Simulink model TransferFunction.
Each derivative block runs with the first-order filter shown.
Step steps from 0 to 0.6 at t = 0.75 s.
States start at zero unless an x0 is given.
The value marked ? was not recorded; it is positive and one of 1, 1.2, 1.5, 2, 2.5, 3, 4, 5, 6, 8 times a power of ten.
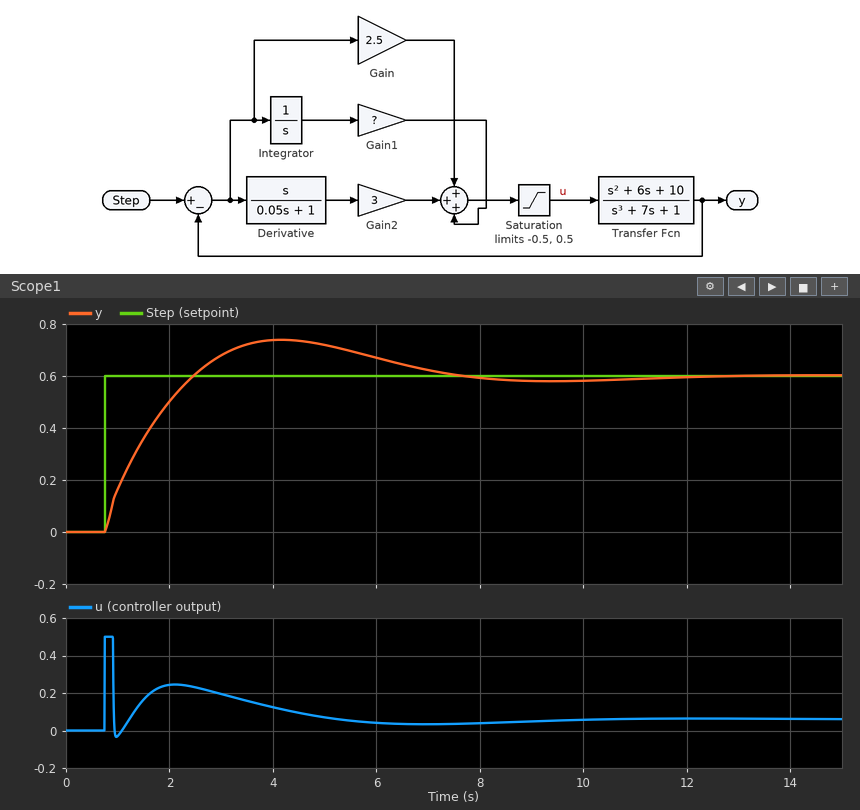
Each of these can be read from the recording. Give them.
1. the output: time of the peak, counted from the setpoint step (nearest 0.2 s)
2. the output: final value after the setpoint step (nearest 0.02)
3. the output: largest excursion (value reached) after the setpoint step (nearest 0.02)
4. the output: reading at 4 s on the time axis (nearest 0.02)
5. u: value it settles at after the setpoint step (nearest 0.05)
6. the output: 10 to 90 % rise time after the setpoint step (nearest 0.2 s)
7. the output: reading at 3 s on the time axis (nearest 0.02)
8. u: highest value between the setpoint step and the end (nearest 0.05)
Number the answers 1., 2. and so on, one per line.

1. 3.4 s
2. 0.60
3. 0.74
4. 0.74
5. 0.05
6. 1.4 s
7. 0.68
8. 0.50
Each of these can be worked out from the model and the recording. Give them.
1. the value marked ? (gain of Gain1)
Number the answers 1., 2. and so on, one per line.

1. 2
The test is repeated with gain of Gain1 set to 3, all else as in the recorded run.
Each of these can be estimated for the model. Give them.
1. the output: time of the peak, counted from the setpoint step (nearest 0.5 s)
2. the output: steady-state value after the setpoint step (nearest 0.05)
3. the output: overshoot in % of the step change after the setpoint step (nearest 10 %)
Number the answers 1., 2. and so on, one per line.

1. 3.0 s
2. 0.60
3. 30 %
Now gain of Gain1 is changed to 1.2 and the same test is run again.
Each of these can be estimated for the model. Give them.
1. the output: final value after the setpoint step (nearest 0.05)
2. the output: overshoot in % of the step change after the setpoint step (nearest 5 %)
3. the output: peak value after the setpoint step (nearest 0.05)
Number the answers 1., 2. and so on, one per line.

1. 0.60
2. 20 %
3. 0.70
